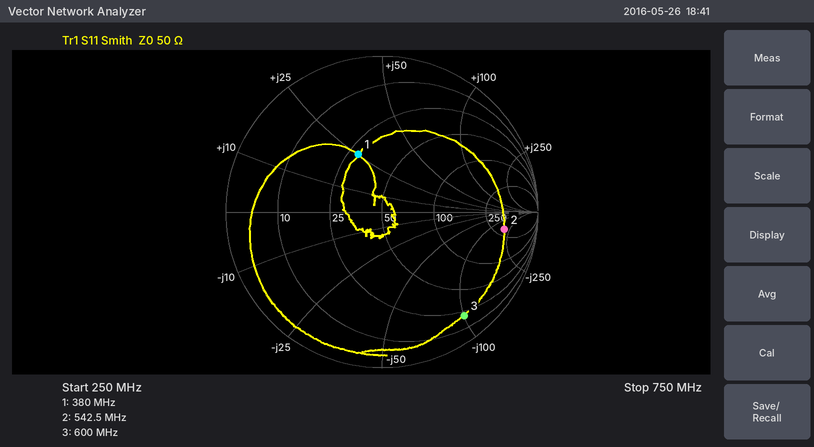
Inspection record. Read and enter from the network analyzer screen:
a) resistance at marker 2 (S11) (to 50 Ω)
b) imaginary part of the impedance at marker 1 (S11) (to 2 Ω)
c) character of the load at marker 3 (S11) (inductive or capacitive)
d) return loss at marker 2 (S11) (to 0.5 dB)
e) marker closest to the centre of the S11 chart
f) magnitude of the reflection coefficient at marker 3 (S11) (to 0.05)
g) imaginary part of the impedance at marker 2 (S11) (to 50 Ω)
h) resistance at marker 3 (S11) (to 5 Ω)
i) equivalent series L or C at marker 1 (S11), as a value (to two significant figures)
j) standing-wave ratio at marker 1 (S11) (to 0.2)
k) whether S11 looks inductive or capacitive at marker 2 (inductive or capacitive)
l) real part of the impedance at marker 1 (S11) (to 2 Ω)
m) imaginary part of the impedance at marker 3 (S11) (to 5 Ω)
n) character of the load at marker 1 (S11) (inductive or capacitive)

300 Ω
+26 Ω
capacitive
2.0 dB
marker 1
0.85
-200 Ω
20 Ω
11 nH
2.4
capacitive
28 Ω
-100 Ω
inductive
